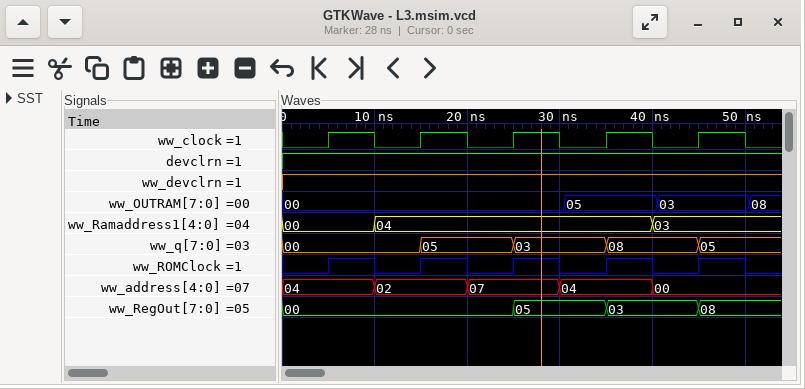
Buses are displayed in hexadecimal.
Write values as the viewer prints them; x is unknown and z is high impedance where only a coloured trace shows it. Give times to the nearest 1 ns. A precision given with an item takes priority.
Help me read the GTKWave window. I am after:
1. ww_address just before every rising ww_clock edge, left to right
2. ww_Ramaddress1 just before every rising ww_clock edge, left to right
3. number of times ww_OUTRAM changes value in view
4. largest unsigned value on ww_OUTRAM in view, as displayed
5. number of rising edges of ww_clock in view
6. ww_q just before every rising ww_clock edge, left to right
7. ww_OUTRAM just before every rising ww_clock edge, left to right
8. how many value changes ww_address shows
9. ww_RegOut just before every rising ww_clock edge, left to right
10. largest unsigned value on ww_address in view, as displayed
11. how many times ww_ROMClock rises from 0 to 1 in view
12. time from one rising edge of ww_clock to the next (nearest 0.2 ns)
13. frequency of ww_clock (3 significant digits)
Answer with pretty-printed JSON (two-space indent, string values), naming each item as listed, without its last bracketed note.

{
  "ww_address just before every rising ww_clock edge, left to right": "04, 02, 07, 04, 00",
  "ww_Ramaddress1 just before every rising ww_clock edge, left to right": "00, 04, 04, 04, 03",
  "number of times ww_OUTRAM changes value in view": "3",
  "largest unsigned value on ww_OUTRAM in view, as displayed": "08",
  "number of rising edges of ww_clock in view": "5",
  "ww_q just before every rising ww_clock edge, left to right": "00, 00, 05, 03, 08",
  "ww_OUTRAM just before every rising ww_clock edge, left to right": "00, 00, 00, 05, 03",
  "how many value changes ww_address shows": "4",
  "ww_RegOut just before every rising ww_clock edge, left to right": "00, 00, 00, 05, 03",
  "largest unsigned value on ww_address in view, as displayed": "07",
  "how many times ww_ROMClock rises from 0 to 1 in view": "5",
  "time from one rising edge of ww_clock to the next": "10 ns",
  "frequency of ww_clock": "100 MHz"
}
